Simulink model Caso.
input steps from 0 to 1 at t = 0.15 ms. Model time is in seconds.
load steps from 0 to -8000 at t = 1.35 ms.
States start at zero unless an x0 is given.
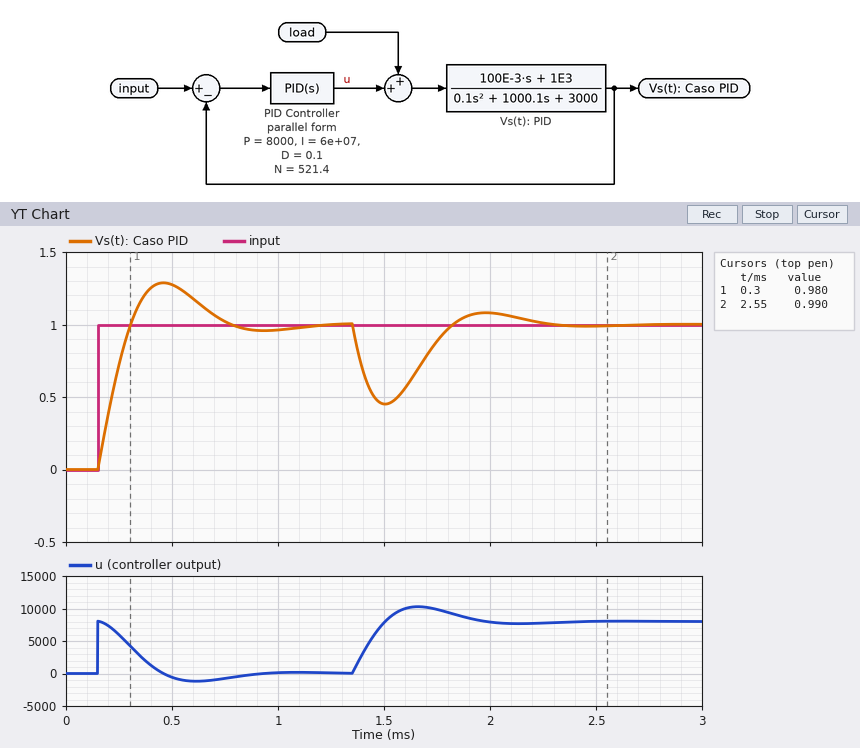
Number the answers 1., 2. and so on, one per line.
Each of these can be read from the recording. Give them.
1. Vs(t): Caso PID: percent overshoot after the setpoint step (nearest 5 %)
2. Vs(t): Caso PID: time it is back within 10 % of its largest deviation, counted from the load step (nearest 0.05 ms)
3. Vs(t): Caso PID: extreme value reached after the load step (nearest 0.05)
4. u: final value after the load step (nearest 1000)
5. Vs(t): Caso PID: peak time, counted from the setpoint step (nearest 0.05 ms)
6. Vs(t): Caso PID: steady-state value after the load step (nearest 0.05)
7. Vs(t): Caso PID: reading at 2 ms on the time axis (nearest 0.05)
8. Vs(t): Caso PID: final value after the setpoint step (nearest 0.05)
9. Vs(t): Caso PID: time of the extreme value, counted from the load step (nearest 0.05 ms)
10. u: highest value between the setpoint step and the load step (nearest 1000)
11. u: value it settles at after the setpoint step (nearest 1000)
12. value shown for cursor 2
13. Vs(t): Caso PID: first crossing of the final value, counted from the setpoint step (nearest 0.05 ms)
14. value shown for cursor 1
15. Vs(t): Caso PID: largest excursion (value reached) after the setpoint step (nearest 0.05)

1. 30 %
2. 0.75 ms
3. 0.45
4. 8000
5. 0.30 ms
6. 1.00
7. 1.10
8. 1.00
9. 0.15 ms
10. 8000
11. 0
12. 0.990
13. 0.15 ms
14. 0.980
15. 1.30
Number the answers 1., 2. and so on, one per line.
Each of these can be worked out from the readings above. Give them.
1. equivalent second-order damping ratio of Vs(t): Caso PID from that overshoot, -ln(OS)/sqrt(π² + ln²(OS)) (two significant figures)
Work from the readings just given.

1. 0.36
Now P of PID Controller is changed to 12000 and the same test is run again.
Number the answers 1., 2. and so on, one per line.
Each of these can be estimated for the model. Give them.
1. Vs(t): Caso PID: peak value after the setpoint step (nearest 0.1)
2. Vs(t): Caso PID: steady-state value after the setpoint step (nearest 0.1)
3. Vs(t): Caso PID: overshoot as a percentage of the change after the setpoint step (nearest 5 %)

1. 1.2
2. 1.0
3. 20 %
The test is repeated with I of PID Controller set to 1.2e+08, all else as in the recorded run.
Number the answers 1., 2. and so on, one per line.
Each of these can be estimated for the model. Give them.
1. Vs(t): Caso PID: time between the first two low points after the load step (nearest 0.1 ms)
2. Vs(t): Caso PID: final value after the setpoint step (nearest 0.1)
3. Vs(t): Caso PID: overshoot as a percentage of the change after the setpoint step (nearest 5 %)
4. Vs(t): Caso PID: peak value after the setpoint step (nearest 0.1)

1. 0.6 ms
2. 1.0
3. 40 %
4. 1.4
